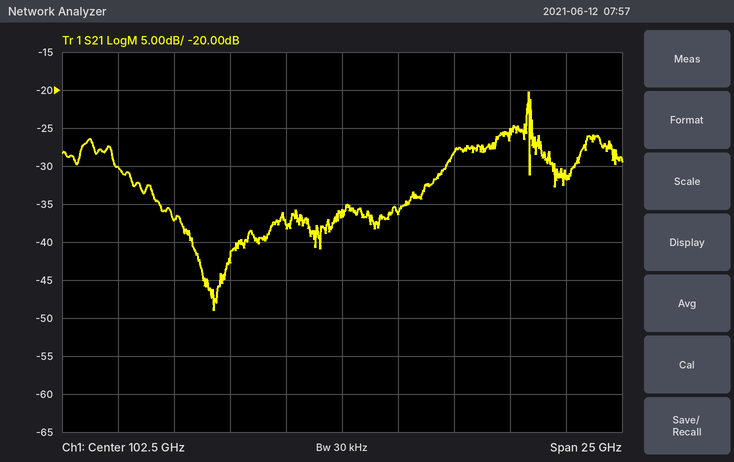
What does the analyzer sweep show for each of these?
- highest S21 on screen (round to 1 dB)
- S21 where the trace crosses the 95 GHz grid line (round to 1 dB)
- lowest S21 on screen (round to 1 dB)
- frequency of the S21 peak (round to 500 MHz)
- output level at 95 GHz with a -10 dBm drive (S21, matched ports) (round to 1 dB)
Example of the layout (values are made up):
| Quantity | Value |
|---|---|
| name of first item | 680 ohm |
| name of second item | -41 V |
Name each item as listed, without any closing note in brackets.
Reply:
| Quantity | Value |
|---|---|
| highest S21 on screen | -20 dB |
| S21 where the trace crosses the 95 GHz grid line | -37 dB |
| lowest S21 on screen | -49 dB |
| frequency of the S21 peak | 111.0 GHz |
| output level at 95 GHz with a -10 dBm drive (S21, matched ports) | -47 dBm |
